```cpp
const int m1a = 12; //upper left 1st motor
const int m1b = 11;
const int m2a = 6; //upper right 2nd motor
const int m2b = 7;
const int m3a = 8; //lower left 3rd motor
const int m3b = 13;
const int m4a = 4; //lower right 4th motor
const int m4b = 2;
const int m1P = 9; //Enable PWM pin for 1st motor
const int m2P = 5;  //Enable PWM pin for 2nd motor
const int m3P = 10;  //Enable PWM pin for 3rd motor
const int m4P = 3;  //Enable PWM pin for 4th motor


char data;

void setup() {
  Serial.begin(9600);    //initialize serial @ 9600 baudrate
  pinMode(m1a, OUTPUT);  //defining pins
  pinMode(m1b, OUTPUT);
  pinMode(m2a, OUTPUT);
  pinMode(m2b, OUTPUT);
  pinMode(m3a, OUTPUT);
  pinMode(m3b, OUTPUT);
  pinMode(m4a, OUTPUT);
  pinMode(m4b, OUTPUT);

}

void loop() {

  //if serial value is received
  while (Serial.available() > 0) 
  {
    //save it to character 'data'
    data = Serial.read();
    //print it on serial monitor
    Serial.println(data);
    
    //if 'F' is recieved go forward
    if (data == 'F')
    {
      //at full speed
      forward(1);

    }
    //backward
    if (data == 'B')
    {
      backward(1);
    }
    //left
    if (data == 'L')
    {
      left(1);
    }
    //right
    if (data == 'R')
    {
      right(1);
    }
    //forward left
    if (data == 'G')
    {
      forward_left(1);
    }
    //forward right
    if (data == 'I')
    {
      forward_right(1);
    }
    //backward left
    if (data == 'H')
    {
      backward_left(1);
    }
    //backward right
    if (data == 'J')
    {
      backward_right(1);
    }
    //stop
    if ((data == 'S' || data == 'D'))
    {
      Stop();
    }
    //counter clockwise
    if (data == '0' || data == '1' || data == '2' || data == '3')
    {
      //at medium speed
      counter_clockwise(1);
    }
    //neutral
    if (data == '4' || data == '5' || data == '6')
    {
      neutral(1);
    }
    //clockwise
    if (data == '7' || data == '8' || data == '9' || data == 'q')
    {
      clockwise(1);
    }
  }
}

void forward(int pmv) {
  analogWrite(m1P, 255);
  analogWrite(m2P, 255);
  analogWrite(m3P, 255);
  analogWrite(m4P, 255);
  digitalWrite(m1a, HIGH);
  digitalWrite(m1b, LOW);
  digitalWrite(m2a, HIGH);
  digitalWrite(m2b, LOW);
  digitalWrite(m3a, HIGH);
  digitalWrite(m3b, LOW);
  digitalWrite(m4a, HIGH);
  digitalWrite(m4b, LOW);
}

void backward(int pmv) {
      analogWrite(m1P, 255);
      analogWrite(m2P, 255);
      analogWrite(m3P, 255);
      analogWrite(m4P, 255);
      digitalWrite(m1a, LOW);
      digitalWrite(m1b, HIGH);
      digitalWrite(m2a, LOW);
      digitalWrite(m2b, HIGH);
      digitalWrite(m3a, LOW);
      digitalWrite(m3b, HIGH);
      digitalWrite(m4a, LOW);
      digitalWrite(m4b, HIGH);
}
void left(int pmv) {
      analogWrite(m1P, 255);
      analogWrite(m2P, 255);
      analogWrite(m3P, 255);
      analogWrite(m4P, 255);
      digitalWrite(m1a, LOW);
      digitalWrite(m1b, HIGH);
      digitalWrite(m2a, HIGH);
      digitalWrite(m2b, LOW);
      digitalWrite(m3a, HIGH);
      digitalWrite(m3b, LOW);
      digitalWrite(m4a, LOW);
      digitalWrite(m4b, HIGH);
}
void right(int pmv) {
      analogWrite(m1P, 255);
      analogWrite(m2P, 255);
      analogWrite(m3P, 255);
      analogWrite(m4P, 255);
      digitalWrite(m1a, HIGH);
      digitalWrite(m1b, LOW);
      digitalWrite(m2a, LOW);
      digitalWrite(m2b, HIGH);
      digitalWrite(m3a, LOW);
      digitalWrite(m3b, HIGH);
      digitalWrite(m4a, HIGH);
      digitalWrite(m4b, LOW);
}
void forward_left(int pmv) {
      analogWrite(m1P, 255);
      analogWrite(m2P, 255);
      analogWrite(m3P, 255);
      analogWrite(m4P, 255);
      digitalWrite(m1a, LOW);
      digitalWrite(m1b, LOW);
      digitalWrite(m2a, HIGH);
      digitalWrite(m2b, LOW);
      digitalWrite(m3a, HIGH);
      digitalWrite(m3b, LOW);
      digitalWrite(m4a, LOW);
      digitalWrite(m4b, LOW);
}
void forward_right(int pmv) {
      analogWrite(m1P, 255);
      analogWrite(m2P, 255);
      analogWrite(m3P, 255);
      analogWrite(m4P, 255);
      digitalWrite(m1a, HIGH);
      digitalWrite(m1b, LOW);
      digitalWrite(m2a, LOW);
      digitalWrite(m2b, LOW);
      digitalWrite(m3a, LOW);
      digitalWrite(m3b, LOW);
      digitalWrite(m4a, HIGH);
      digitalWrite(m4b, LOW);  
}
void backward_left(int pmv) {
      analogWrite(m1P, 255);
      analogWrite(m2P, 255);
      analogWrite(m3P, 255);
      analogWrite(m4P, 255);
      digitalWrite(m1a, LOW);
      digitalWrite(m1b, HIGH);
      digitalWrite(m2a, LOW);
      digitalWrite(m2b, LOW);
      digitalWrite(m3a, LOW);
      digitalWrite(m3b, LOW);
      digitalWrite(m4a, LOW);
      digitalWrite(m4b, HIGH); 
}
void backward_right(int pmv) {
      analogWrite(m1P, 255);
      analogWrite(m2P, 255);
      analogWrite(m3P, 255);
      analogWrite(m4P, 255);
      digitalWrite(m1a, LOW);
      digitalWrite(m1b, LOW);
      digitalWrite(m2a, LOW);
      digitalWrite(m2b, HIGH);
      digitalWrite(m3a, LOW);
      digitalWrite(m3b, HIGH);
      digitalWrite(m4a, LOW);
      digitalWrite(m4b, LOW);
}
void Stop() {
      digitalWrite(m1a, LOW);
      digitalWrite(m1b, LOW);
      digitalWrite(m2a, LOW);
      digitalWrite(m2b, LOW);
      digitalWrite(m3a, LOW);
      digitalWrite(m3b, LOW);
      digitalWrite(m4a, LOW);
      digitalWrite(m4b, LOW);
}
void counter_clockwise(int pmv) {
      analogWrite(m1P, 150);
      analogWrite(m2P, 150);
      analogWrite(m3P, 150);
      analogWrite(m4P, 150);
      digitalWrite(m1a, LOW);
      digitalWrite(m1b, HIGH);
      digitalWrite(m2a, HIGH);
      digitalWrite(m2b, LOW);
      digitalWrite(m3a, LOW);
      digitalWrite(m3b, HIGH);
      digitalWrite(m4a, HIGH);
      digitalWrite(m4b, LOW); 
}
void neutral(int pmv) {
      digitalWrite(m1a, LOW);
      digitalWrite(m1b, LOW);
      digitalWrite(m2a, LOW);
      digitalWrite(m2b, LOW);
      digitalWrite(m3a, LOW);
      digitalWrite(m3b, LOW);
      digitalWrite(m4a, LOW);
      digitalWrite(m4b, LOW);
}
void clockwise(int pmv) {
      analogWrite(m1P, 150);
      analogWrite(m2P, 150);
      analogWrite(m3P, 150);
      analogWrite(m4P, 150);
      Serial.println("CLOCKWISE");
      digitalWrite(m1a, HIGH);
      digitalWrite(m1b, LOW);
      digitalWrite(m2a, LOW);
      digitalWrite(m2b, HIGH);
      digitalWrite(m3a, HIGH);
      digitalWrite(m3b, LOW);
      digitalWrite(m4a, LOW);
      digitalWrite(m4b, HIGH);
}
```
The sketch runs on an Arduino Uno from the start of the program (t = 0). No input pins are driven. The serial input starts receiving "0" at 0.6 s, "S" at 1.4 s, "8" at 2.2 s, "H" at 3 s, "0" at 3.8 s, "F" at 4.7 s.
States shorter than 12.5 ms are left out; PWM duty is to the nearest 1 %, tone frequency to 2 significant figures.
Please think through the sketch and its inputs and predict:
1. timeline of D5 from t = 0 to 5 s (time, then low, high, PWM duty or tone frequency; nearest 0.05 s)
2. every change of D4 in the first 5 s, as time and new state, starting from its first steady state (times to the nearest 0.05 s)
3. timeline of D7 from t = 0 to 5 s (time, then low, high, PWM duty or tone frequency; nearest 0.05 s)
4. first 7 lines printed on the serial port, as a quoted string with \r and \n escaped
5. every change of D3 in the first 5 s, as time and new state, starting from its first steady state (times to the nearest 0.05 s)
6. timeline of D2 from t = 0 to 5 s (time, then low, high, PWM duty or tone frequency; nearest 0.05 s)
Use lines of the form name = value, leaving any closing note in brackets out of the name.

timeline of D5 from t = 0 to 5 s = 0.6 s PWM 59 %; 3 s high; 3.8 s PWM 59 %; 4.7 s high
every change of D4 in the first 5 s, as time and new state, starting from its first steady state = 0 s low; 0.6 s high; 1.4 s low; 3.8 s high
timeline of D7 from t = 0 to 5 s = 0 s low; 2.2 s high; 3 s low
first 7 lines printed on the serial port, as a quoted string with \r and \n escaped = "0\r\nS\r\n8\r\nCLOCKWISE\r\nH\r\n0\r\nF\r\n"
every change of D3 in the first 5 s, as time and new state, starting from its first steady state = 0.6 s PWM 59 %; 3 s high; 3.8 s PWM 59 %; 4.7 s high
timeline of D2 from t = 0 to 5 s = 0 s low; 2.2 s high; 3.8 s low
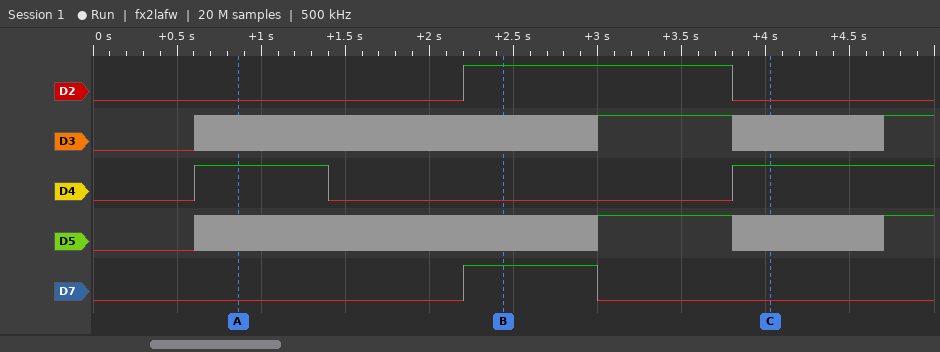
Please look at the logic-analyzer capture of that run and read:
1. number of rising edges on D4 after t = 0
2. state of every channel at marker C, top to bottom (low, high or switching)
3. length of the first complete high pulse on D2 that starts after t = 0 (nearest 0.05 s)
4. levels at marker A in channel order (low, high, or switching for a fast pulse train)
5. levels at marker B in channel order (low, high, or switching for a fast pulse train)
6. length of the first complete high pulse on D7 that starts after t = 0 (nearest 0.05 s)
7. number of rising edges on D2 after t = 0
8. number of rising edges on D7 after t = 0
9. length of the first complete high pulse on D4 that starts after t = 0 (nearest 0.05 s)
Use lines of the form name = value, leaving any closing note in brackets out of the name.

number of rising edges on D4 after t = 0 = 2
state of every channel at marker C, top to bottom = D2 low, D3 switching, D4 high, D5 switching, D7 low
length of the first complete high pulse on D2 that starts after t = 0 = 1.60 s
levels at marker A in channel order = D2 low, D3 switching, D4 high, D5 switching, D7 low
levels at marker B in channel order = D2 high, D3 switching, D4 low, D5 switching, D7 high
length of the first complete high pulse on D7 that starts after t = 0 = 0.80 s
number of rising edges on D2 after t = 0 = 1
number of rising edges on D7 after t = 0 = 1
length of the first complete high pulse on D4 that starts after t = 0 = 0.80 s
